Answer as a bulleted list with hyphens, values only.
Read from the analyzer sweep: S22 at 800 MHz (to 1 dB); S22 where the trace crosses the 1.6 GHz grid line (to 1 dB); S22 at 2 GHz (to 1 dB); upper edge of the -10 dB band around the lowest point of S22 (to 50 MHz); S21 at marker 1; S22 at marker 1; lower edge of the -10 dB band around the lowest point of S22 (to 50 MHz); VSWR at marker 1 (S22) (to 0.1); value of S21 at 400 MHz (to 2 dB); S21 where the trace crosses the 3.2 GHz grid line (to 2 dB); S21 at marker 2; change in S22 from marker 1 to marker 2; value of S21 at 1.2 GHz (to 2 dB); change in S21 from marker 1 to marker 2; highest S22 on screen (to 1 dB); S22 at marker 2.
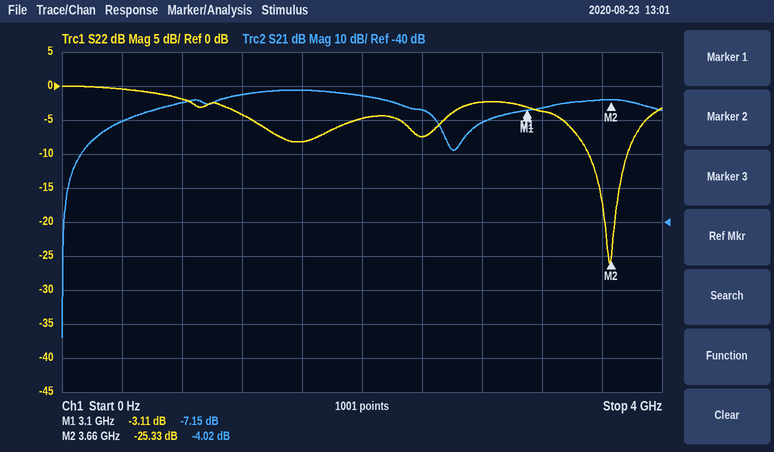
- -2 dB
- -8 dB
- -5 dB
- 3.75 GHz
- -7.15 dB
- -3.11 dB
- 3.50 GHz
- 5.6
- -10 dB
- -6 dB
- -4.02 dB
- -22.22 dB
- -2 dB
- 3.13 dB
- 0 dB
- -25.33 dB
